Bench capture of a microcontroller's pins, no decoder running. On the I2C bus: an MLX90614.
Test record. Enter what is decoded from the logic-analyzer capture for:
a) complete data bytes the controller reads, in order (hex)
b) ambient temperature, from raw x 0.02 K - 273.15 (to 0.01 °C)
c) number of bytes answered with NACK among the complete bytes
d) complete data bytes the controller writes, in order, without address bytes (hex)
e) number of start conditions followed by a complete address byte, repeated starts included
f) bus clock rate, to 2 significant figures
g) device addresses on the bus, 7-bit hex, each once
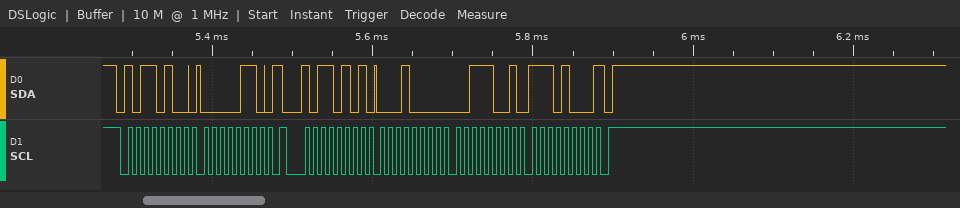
10 39 E8
19.01 °C
1
06
2
100 kHz
0x5A
